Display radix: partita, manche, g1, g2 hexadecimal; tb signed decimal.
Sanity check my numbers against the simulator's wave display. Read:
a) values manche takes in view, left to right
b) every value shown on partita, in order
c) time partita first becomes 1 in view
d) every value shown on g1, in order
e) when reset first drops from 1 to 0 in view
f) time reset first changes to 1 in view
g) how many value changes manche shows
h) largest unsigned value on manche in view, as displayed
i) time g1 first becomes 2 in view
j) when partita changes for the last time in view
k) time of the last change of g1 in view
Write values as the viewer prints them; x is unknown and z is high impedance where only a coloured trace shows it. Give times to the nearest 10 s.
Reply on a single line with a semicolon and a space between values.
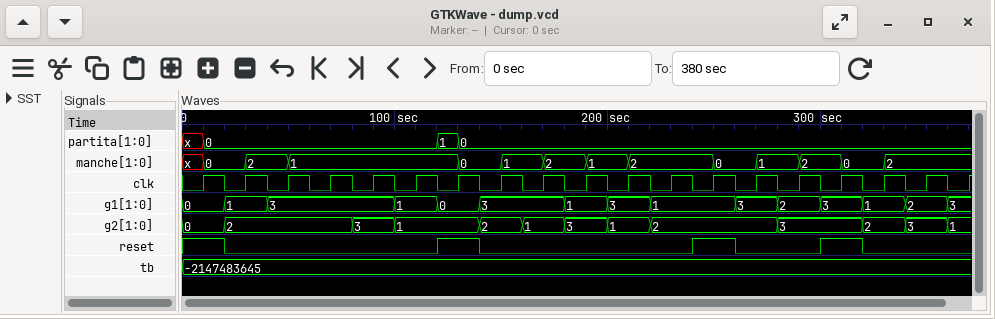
x, 0, 2, 1, 0, 1, 2, 1, 2, 0, 1, 2, 0, 2; x, 0, 1, 0; 120 s; 0, 1, 3, 1, 0, 3, 1, 3, 1, 3, 2, 3, 1, 2, 3; 20 s; 120 s; 13; 2; 280 s; 130 s; 360 s
